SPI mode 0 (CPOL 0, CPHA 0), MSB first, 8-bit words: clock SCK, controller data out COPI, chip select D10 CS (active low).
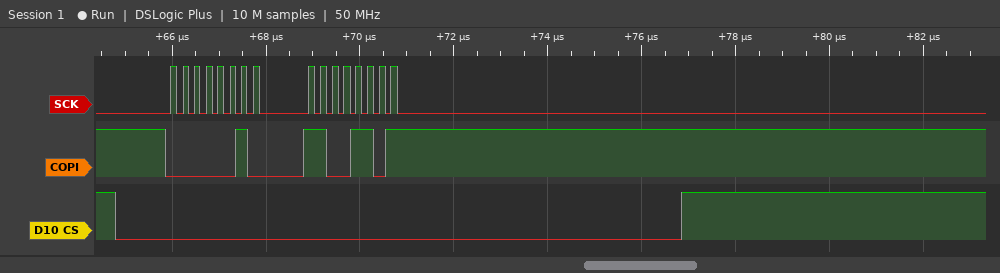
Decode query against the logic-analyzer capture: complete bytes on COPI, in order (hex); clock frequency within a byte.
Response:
0x02 0xCD
4 MHz
